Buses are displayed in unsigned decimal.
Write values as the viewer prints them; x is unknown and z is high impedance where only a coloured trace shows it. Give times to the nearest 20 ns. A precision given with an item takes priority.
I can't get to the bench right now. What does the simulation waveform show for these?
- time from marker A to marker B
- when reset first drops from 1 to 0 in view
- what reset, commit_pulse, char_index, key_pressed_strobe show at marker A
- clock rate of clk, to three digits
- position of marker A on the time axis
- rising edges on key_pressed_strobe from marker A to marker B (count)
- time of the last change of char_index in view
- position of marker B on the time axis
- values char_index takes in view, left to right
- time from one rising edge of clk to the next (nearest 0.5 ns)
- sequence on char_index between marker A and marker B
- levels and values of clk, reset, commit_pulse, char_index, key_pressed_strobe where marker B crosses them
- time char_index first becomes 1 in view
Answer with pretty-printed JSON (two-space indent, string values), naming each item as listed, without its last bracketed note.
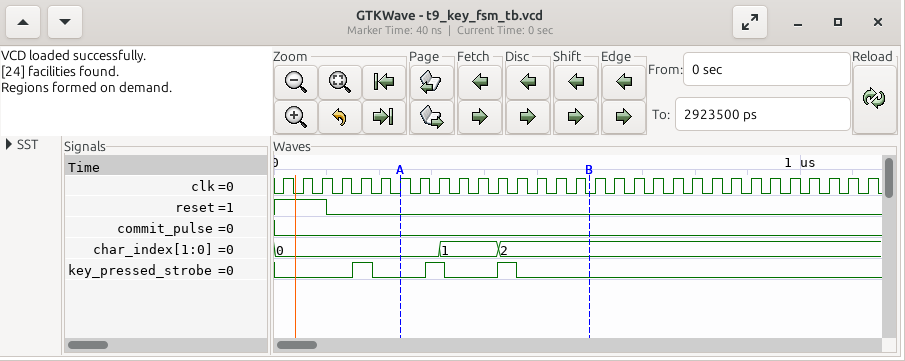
{
  "time from marker A to marker B": "360 ns",
  "when reset first drops from 1 to 0 in view": "100 ns",
  "what reset, commit_pulse, char_index, key_pressed_strobe show at marker A": "reset=0, commit_pulse=0, char_index=0, key_pressed_strobe=0",
  "clock rate of clk, to three digits": "27.0 MHz",
  "position of marker A on the time axis": "240 ns",
  "rising edges on key_pressed_strobe from marker A to marker B": "2",
  "time of the last change of char_index in view": "420 ns",
  "position of marker B on the time axis": "600 ns",
  "values char_index takes in view, left to right": "0, 1, 2",
  "time from one rising edge of clk to the next": "37 ns",
  "sequence on char_index between marker A and marker B": "0, 1, 2",
  "levels and values of clk, reset, commit_pulse, char_index, key_pressed_strobe where marker B crosses them": "clk=0, reset=0, commit_pulse=0, char_index=2, key_pressed_strobe=0",
  "time char_index first becomes 1 in view": "320 ns"
}
